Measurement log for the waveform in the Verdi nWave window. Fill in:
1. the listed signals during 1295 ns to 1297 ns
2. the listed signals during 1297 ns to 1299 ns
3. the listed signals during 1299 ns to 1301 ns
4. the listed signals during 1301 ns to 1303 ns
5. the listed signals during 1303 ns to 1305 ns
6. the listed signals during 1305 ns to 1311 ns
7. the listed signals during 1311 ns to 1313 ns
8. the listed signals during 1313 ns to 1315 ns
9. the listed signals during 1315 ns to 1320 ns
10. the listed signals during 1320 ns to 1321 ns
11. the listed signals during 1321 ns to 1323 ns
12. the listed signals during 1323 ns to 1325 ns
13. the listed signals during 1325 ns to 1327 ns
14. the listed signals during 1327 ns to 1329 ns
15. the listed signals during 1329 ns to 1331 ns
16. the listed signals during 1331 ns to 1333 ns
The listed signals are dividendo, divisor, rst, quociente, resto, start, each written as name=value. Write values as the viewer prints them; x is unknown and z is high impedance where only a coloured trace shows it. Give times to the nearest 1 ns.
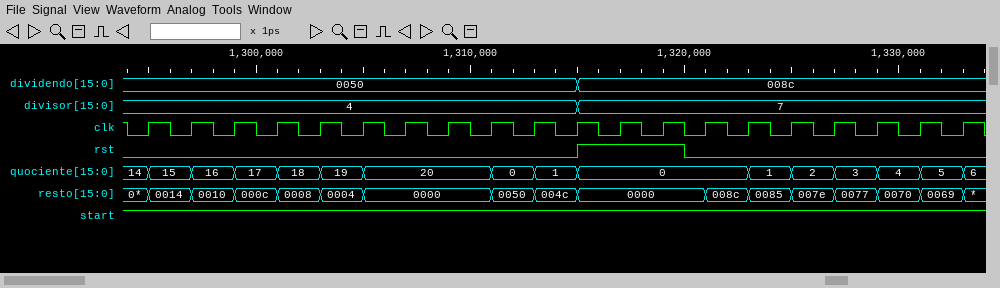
dividendo=0050, divisor=4, rst=0, quociente=15, resto=0014, start=1
dividendo=0050, divisor=4, rst=0, quociente=16, resto=0010, start=1
dividendo=0050, divisor=4, rst=0, quociente=17, resto=000c, start=1
dividendo=0050, divisor=4, rst=0, quociente=18, resto=0008, start=1
dividendo=0050, divisor=4, rst=0, quociente=19, resto=0004, start=1
dividendo=0050, divisor=4, rst=0, quociente=20, resto=0000, start=1
dividendo=0050, divisor=4, rst=0, quociente=0, resto=0050, start=1
dividendo=0050, divisor=4, rst=0, quociente=1, resto=004c, start=1
dividendo=008c, divisor=7, rst=1, quociente=0, resto=0000, start=1
dividendo=008c, divisor=7, rst=0, quociente=0, resto=0000, start=1
dividendo=008c, divisor=7, rst=0, quociente=0, resto=008c, start=1
dividendo=008c, divisor=7, rst=0, quociente=1, resto=0085, start=1
dividendo=008c, divisor=7, rst=0, quociente=2, resto=007e, start=1
dividendo=008c, divisor=7, rst=0, quociente=3, resto=0077, start=1
dividendo=008c, divisor=7, rst=0, quociente=4, resto=0070, start=1
dividendo=008c, divisor=7, rst=0, quociente=5, resto=0069, start=1
